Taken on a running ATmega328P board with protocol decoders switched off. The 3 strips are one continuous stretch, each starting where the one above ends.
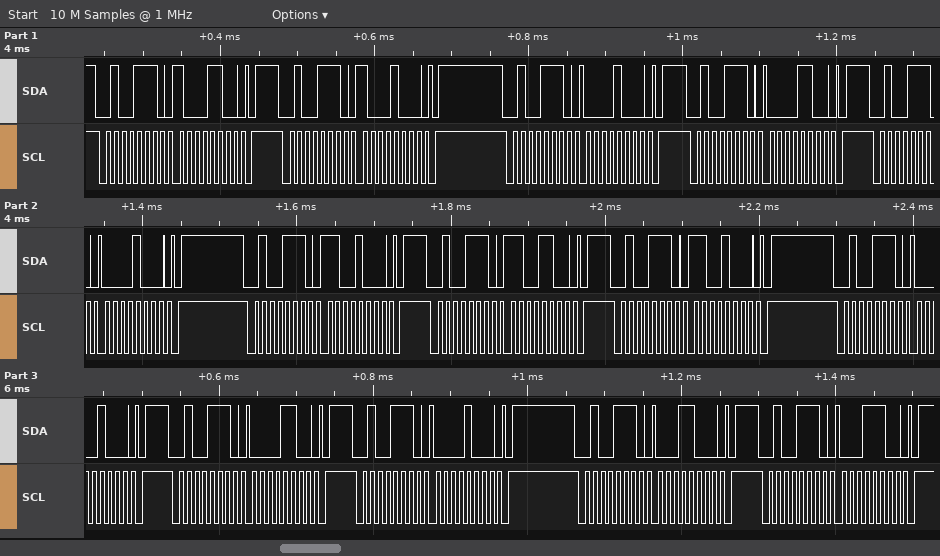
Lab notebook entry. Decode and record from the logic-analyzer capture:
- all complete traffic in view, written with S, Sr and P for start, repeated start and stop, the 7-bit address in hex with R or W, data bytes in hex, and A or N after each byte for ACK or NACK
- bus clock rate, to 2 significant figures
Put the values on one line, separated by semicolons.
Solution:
S 27W A 8C A P S 27W A 88 A P S 27W A 08 A P S 27W A 0C A P S 27W A 08 A P S 27W A C8 A P S 27W A CC A P S 27W A C8 A P S 27W A 08 A P S 27W A 0C A P S 27W A 08 A P S 27W A 18 A P S 27W A 1C A P; 100 kHz
